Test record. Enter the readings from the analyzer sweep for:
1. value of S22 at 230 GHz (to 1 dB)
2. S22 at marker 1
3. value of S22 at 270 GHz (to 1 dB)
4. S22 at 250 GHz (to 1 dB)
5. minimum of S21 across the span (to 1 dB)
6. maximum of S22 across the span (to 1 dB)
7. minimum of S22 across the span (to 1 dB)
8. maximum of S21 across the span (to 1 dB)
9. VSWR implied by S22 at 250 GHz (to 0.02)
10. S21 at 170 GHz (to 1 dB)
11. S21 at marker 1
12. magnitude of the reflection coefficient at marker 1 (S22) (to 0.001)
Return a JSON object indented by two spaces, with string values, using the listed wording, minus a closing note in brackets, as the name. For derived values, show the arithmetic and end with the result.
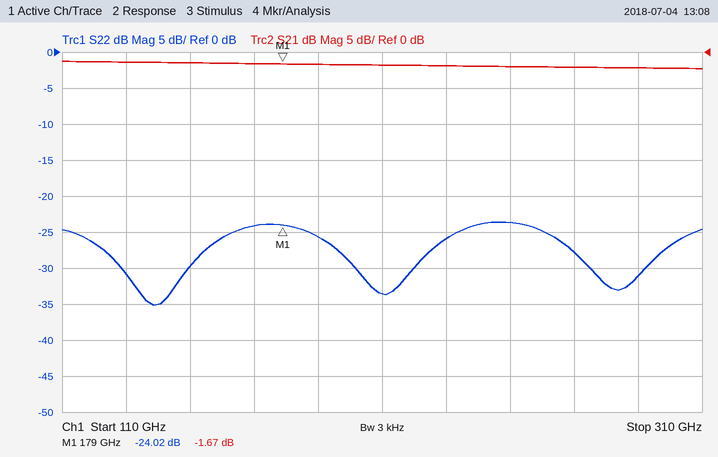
{
  "value of S22 at 230 GHz": "-26 dB",
  "S22 at marker 1": "-24.02 dB",
  "value of S22 at 270 GHz": "-28 dB",
  "S22 at 250 GHz": "-24 dB",
  "minimum of S21 across the span": "-2 dB",
  "maximum of S22 across the span": "-24 dB",
  "minimum of S22 across the span": "-35 dB",
  "maximum of S21 across the span": "-1 dB",
  "VSWR implied by S22 at 250 GHz": "|Γ| = 10^(-24/20) = 0.0631; VSWR = (1 + 0.0631)/(1 − 0.0631) ≈ 1.13, so 1.14 to the nearest 0.02",
  "S21 at 170 GHz": "-2 dB",
  "S21 at marker 1": "-1.67 dB",
  "magnitude of the reflection coefficient at marker 1 (S22)": "10^(-24.02/20) ≈ 0.063"
}
